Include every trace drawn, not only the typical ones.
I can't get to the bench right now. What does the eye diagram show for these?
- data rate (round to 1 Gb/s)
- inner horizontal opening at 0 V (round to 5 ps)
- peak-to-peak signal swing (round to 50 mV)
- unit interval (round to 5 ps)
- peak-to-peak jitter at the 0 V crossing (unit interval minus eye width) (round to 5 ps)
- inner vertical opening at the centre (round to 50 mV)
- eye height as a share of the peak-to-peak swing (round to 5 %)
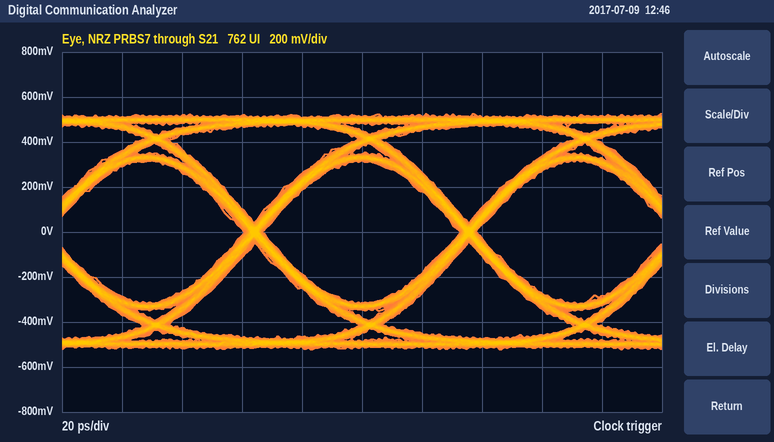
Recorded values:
14 Gb/s
65 ps
1.05 V
70 ps
5 ps
650 mV
60 %
